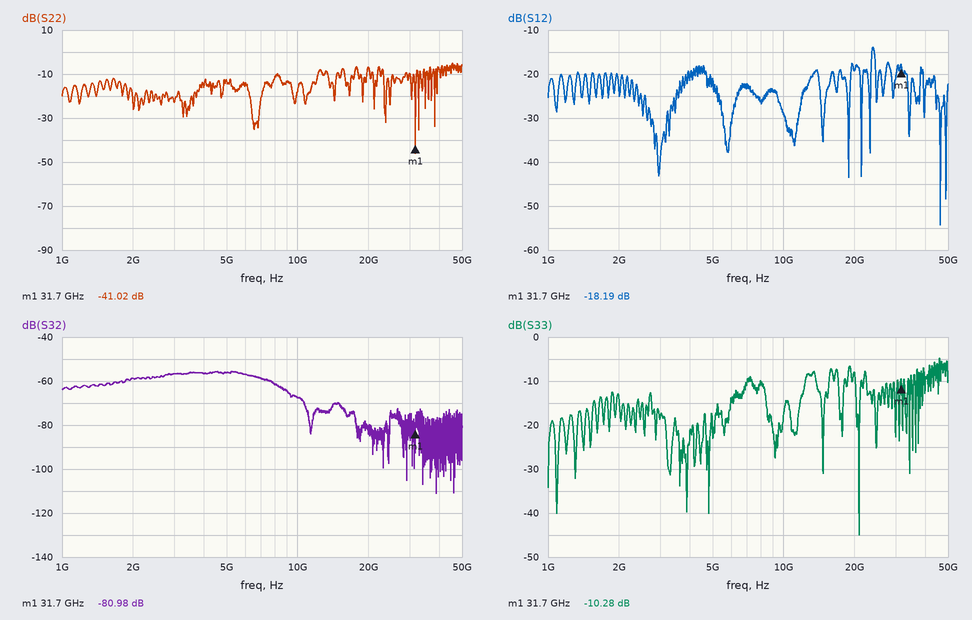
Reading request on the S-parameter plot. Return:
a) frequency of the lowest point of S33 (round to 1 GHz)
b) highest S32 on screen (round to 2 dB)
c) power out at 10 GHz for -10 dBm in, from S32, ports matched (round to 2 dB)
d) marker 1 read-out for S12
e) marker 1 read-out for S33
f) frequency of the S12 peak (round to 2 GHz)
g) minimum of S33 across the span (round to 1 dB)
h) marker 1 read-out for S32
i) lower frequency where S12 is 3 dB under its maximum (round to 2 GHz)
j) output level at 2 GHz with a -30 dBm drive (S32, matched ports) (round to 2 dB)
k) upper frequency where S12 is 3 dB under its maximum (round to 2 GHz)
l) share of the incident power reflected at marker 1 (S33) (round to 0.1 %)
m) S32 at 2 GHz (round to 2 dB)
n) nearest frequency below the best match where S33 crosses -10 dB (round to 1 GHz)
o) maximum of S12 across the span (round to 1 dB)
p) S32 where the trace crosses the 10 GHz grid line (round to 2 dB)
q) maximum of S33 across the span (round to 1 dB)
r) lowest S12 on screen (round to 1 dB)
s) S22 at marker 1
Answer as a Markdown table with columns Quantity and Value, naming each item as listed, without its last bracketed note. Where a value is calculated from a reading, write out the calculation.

| Quantity | Value |
|---|---|
| frequency of the lowest point of S33 | 21 GHz |
| highest S32 on screen | -56 dB |
| power out at 10 GHz for -10 dBm in, from S32, ports matched | -10 dBm + (-68 dB) = -78 dBm |
| marker 1 read-out for S12 | -18.19 dB |
| marker 1 read-out for S33 | -10.28 dB |
| frequency of the S12 peak | 24 GHz |
| minimum of S33 across the span | -45 dB |
| marker 1 read-out for S32 | -80.98 dB |
| lower frequency where S12 is 3 dB under its maximum | 24 GHz |
| output level at 2 GHz with a -30 dBm drive (S32, matched ports) | -30 dBm + (-58 dB) = -88 dBm |
| upper frequency where S12 is 3 dB under its maximum | 24 GHz |
| share of the incident power reflected at marker 1 (S33) | 10^(-10.28/10) ≈ 9.4 % |
| S32 at 2 GHz | -58 dB |
| nearest frequency below the best match where S33 crosses -10 dB | 20 GHz |
| maximum of S12 across the span | -14 dB |
| S32 where the trace crosses the 10 GHz grid line | -68 dB |
| maximum of S33 across the span | -5 dB |
| lowest S12 on screen | -54 dB |
| S22 at marker 1 | -41.02 dB |
